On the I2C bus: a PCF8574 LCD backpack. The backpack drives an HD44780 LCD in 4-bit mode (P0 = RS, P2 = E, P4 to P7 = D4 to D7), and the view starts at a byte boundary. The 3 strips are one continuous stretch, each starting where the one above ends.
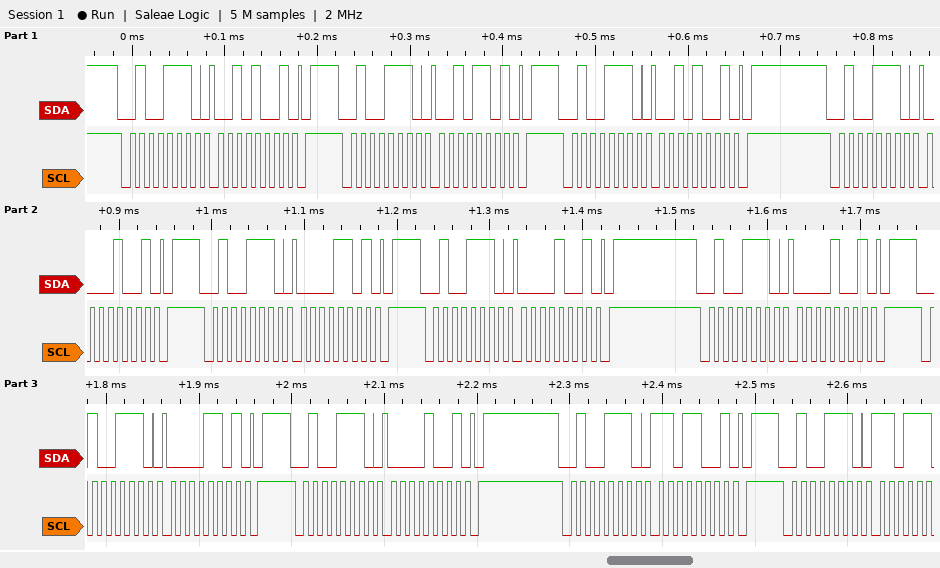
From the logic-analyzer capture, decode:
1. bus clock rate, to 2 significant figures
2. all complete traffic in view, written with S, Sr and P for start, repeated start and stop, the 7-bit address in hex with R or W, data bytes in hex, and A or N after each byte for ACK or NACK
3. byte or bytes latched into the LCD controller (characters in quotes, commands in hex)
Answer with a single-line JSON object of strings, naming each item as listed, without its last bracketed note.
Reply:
{"bus clock rate, to 2 significant figures": "100 kHz", "all complete traffic in view, written with S, Sr and P for start, repeated start and stop, the 7-bit address in hex with R or W, data bytes in hex, and A or N after each byte for ACK or NACK": "S 27W A 29 A P S 27W A 2D A P S 27W A 29 A P S 27W A 09 A P S 27W A 0D A P S 27W A 09 A P S 27W A 09 A P S 27W A 0D A P S 27W A 09 A P S 27W A D9 A P S 27W A", "byte or bytes latched into the LCD controller": "' '"}
